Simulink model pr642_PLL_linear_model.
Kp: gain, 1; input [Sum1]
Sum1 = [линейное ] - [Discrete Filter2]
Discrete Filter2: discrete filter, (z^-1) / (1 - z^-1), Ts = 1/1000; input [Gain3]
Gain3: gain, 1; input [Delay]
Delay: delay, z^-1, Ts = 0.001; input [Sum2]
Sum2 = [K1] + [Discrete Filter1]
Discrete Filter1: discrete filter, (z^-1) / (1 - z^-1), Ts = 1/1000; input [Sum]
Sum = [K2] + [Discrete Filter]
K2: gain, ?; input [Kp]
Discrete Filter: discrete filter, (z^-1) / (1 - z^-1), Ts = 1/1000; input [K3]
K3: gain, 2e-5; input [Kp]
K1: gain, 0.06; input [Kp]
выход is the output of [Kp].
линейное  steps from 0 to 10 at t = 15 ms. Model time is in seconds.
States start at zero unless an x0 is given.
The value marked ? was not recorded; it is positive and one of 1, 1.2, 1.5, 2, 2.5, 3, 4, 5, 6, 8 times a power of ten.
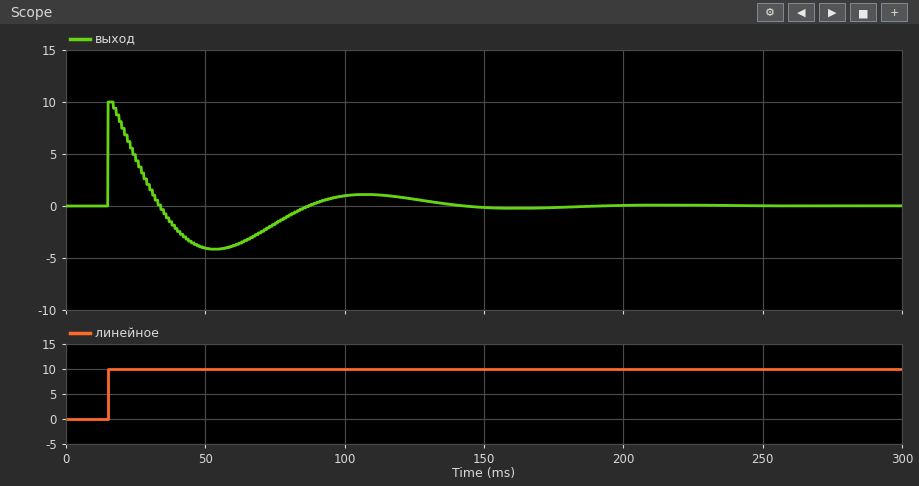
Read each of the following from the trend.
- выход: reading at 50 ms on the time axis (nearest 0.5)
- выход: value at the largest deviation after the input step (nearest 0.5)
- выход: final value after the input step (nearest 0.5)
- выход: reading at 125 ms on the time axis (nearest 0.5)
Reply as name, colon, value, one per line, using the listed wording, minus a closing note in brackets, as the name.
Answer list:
выход: reading at 50 ms on the time axis: -4.0
выход: value at the largest deviation after the input step: 10.0
выход: final value after the input step: 0.0
выход: reading at 125 ms on the time axis: 0.5
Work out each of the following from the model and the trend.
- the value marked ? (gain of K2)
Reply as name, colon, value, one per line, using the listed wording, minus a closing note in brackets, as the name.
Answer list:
the value marked ?: 0.004
